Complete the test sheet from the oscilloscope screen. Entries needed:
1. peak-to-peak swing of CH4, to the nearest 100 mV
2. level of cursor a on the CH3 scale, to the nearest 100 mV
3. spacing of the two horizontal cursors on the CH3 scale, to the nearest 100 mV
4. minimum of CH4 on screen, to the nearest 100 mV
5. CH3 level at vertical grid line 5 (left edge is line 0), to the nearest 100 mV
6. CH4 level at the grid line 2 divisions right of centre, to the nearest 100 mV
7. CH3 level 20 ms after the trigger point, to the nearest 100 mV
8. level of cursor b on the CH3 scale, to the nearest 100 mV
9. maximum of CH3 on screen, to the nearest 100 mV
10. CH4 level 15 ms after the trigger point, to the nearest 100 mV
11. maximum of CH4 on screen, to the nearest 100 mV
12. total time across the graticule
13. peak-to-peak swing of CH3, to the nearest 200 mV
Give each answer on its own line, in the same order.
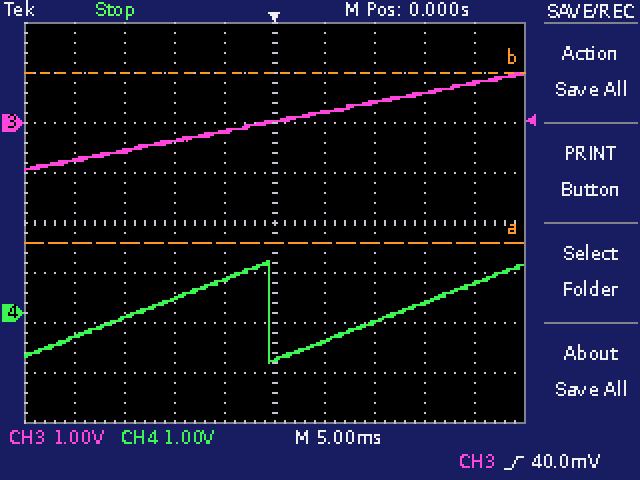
2.0 V
-2.4 V
3.4 V
-1.0 V
0.0 V
-200 mV
800 mV
1.0 V
1.0 V
200 mV
1.0 V
50 ms
2.0 V
